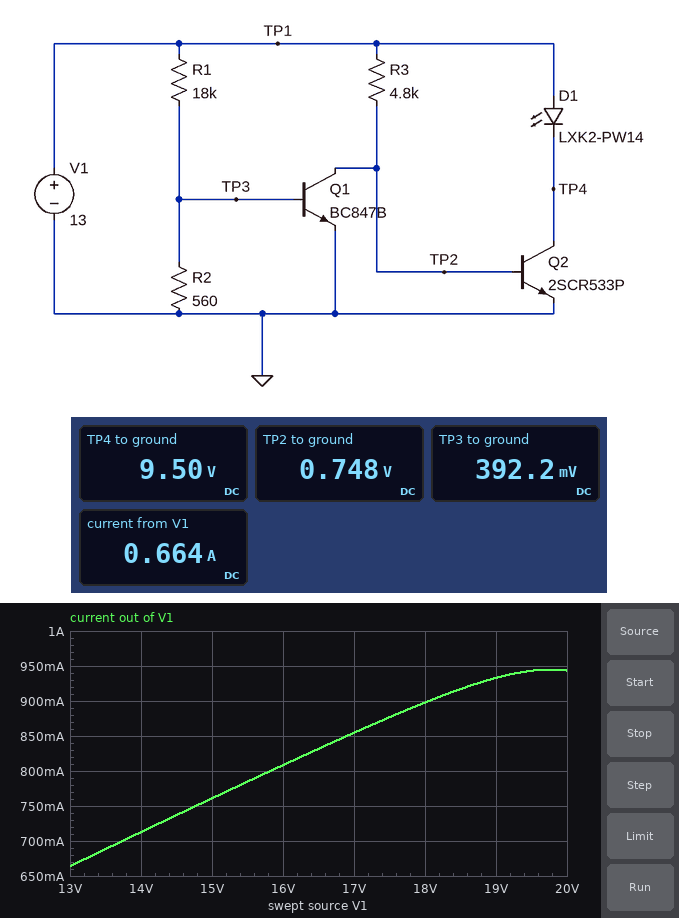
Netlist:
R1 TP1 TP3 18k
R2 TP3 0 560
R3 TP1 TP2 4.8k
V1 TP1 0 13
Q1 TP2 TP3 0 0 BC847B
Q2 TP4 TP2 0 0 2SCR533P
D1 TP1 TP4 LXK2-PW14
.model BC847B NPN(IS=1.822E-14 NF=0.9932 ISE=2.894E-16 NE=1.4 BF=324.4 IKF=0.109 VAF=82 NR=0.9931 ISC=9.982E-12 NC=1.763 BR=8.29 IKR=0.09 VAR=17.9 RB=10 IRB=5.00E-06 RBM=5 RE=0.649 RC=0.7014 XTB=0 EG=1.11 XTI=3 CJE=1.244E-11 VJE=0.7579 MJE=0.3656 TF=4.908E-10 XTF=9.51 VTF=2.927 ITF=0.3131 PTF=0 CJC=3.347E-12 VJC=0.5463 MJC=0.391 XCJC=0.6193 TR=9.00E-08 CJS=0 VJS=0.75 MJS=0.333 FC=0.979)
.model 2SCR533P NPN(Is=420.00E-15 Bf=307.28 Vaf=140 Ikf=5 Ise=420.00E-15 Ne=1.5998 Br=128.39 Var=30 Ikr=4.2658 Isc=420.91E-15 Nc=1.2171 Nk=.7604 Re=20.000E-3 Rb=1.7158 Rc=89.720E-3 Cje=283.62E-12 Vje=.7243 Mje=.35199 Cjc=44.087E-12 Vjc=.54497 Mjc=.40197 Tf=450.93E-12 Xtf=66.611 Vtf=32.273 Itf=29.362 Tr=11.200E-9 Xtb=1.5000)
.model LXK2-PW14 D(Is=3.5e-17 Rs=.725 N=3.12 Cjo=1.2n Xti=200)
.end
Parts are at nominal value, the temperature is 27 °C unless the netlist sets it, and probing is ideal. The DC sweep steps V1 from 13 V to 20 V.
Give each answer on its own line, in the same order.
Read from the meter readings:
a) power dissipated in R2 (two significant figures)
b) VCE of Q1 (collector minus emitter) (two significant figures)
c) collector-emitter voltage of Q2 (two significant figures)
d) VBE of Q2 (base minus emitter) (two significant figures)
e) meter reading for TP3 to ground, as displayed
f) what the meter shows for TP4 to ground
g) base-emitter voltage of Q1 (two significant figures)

270 µW
750 mV
9.5 V
750 mV
392.2 mV
9.50 V
390 mV
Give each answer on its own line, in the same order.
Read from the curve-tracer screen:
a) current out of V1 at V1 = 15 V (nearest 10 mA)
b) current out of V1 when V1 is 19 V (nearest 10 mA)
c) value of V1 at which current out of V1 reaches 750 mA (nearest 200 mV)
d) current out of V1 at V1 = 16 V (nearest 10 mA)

760 mA
930 mA
14.8 V
810 mA
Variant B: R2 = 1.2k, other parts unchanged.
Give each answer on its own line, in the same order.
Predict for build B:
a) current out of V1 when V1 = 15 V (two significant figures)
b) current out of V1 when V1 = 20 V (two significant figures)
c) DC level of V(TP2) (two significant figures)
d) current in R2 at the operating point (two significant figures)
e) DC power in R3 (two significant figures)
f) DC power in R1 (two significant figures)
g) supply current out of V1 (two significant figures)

3.9 mA
5.2 mA
43 mV
560 µA
35 mW
8.4 mW
3.4 mA
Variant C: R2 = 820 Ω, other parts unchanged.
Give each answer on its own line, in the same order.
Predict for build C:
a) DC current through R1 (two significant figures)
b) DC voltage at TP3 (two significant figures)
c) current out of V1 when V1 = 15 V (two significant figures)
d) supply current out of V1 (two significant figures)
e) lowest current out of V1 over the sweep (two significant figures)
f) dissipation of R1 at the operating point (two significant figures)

690 µA
570 mV
400 mA
650 mA
4.0 mA
8.6 mW
